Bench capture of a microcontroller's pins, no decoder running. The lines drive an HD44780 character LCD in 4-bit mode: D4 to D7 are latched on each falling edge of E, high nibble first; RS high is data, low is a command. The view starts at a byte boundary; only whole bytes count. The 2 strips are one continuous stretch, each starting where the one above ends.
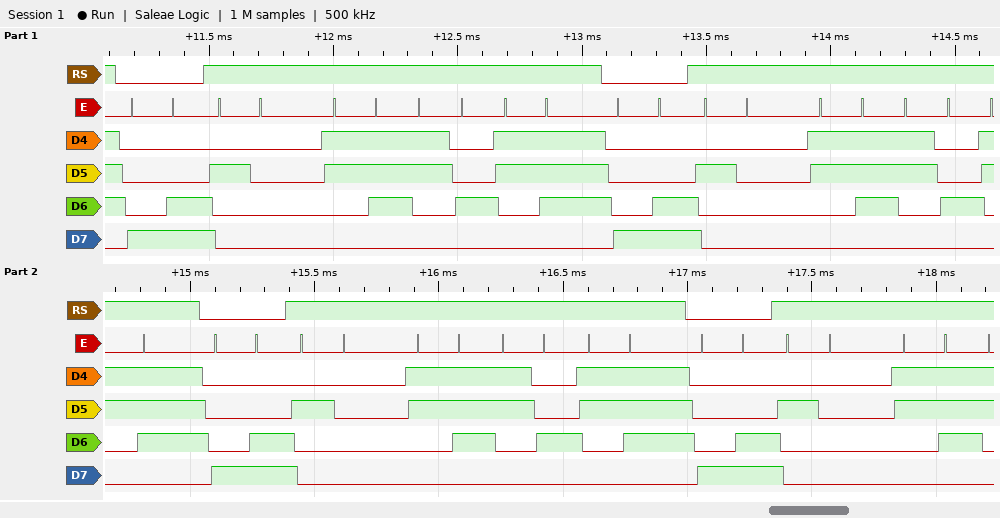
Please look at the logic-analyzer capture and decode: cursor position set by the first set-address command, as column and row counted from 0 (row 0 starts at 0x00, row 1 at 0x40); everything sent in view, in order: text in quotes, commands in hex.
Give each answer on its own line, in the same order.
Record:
column 12, row 0
0x8C " 747" 0x8C " 747" 0x8C " 747" 0x8C " 7"
